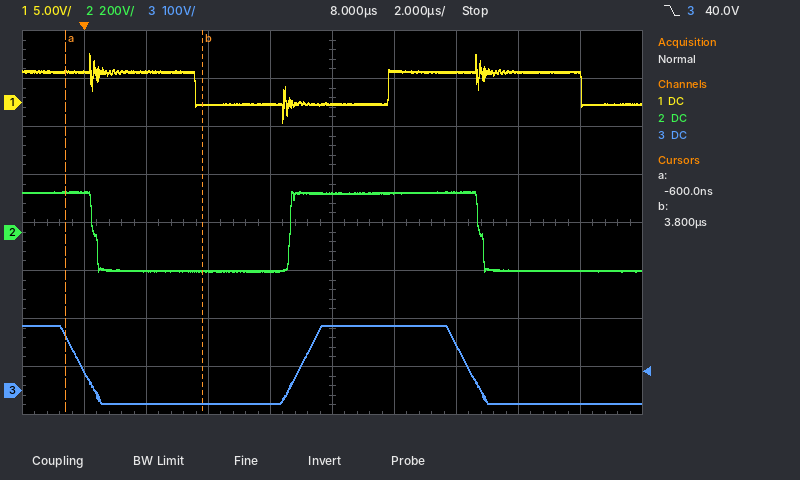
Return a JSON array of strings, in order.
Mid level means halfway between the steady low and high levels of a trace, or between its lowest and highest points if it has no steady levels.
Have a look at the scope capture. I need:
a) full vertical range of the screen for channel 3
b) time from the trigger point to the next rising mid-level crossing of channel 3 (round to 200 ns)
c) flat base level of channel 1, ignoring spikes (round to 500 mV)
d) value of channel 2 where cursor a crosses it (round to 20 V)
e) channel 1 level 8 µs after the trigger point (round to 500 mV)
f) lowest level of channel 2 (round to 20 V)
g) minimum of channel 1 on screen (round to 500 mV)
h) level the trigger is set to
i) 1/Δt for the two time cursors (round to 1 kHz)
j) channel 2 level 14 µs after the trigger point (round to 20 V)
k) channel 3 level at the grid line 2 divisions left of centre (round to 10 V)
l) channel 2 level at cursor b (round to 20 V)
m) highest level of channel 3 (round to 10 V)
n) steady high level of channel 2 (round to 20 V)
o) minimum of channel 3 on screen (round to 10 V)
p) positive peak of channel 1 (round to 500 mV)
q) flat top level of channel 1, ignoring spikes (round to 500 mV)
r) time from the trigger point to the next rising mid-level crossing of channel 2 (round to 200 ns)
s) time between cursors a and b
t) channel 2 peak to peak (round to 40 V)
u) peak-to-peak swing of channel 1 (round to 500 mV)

["800 V", "7.0 µs", "0.0 V", "160 V", "0.0 V", "-160 V", "-2.0 V", "40.0 V", "227 kHz", "-160 V", "-30 V", "-160 V", "140 V", "160 V", "-30 V", "5.0 V", "3.0 V", "6.6 µs", "4.4 µs", "320 V", "7.0 V"]
